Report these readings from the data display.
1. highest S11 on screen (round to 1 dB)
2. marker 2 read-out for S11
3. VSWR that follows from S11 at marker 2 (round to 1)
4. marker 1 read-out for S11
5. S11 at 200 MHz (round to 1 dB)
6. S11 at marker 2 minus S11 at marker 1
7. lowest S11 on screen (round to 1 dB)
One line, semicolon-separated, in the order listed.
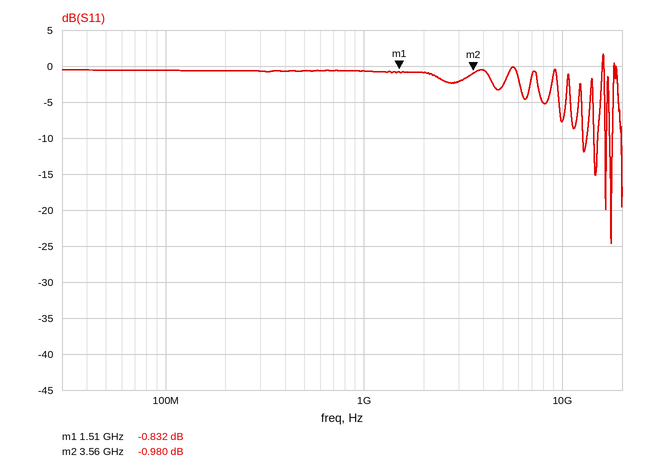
2 dB; -0.980 dB; 18; -0.832 dB; -1 dB; -0.148 dB; -25 dB
